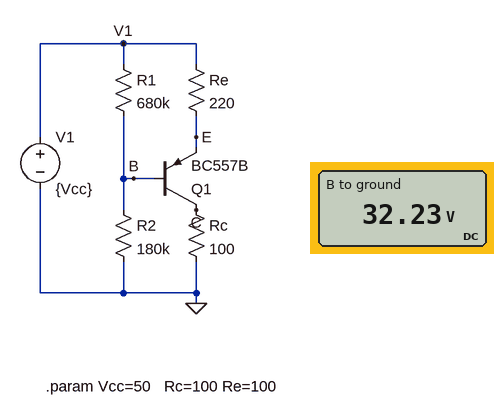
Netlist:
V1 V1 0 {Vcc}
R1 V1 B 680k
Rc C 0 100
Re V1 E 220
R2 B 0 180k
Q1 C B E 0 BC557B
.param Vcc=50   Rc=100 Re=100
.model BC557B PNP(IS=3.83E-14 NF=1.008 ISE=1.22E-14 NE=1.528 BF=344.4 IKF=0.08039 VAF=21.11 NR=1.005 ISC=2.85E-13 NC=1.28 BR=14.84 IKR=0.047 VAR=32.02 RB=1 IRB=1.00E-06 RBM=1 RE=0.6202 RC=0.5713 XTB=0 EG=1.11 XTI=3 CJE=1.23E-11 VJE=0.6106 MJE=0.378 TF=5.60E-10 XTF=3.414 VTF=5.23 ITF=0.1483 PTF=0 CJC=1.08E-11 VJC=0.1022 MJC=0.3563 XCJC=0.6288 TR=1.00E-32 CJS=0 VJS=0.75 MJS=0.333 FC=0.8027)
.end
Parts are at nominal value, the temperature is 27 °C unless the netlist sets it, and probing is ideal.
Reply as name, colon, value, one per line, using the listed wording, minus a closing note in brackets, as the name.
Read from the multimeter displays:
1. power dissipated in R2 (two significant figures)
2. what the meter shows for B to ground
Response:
power dissipated in R2: 5.8 mW
what the meter shows for B to ground: 32.23 V
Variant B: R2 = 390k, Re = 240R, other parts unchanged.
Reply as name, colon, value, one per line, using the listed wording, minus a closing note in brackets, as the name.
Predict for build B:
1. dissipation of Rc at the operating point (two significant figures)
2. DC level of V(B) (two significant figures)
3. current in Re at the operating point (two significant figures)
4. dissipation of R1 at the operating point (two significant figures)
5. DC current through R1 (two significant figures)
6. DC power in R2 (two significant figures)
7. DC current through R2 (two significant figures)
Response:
dissipation of Rc at the operating point: 260 mW
DC level of V(B): 37 V
current in Re at the operating point: 51 mA
dissipation of R1 at the operating point: 250 µW
DC current through R1: 19 µA
DC power in R2: 3.5 mW
DC current through R2: 95 µA
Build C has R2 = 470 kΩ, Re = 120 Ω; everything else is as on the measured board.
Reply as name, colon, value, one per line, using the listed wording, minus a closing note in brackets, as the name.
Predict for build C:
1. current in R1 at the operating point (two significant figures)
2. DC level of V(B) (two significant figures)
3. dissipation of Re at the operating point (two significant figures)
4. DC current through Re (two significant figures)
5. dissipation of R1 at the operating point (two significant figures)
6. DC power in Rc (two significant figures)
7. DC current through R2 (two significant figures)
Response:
current in R1 at the operating point: 11 µA
DC level of V(B): 42 V
dissipation of Re at the operating point: 400 mW
DC current through Re: 58 mA
dissipation of R1 at the operating point: 86 µW
DC power in Rc: 330 mW
DC current through R2: 90 µA
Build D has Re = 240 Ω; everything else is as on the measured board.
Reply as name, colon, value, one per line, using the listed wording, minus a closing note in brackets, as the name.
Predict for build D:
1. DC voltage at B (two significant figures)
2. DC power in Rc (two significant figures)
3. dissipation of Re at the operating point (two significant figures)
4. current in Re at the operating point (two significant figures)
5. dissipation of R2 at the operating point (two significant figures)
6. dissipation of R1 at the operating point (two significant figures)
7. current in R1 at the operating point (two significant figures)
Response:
DC voltage at B: 31 V
DC power in Rc: 550 mW
dissipation of Re at the operating point: 1.3 W
current in Re at the operating point: 74 mA
dissipation of R2 at the operating point: 5.5 mW
dissipation of R1 at the operating point: 510 µW
current in R1 at the operating point: 27 µA
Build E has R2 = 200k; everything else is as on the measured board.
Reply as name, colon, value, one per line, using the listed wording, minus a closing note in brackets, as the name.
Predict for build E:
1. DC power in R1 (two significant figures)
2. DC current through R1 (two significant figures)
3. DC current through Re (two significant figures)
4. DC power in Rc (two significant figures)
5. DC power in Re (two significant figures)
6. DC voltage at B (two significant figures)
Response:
DC power in R1: 430 µW
DC current through R1: 25 µA
DC current through Re: 74 mA
DC power in Rc: 540 mW
DC power in Re: 1.2 W
DC voltage at B: 33 V
